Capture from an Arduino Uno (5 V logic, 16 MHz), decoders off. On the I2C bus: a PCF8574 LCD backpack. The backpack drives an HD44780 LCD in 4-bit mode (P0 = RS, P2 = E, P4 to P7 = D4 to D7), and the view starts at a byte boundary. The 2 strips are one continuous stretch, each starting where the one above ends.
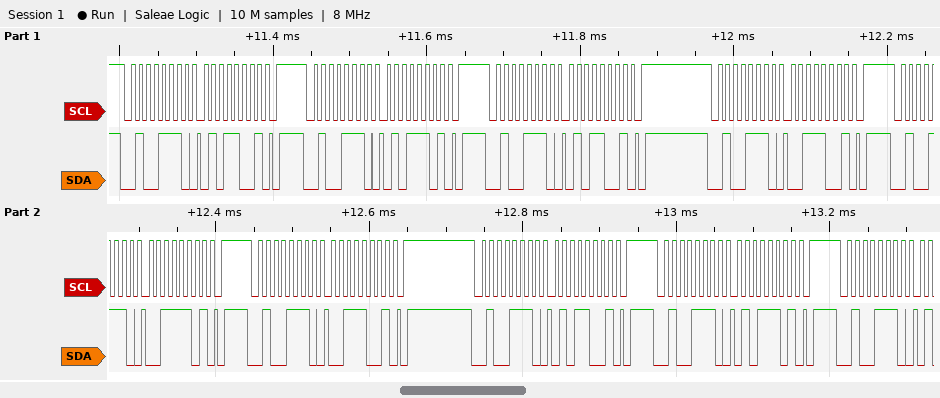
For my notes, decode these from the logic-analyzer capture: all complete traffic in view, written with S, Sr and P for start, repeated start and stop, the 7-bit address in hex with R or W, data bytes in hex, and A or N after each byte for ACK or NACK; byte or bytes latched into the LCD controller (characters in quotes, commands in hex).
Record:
S 27W A 59 A P S 27W A 5D A P S 27W A 59 A P S 27W A 39 A P S 27W A 3D A P S 27W A 39 A P S 27W A 59 A P S 27W A 5D A P S 27W A
'S'
